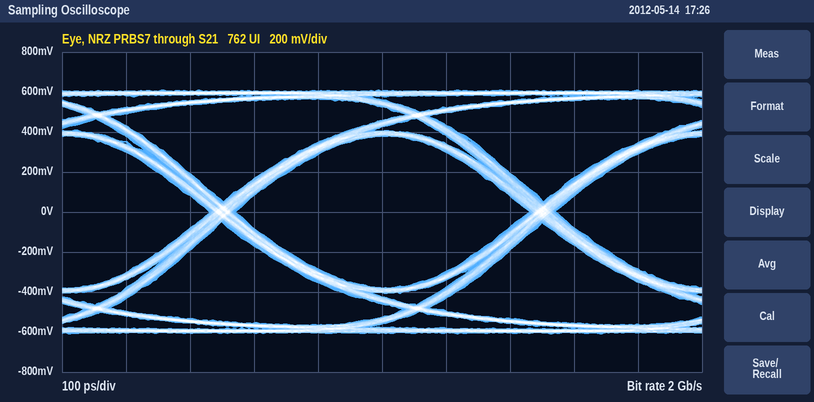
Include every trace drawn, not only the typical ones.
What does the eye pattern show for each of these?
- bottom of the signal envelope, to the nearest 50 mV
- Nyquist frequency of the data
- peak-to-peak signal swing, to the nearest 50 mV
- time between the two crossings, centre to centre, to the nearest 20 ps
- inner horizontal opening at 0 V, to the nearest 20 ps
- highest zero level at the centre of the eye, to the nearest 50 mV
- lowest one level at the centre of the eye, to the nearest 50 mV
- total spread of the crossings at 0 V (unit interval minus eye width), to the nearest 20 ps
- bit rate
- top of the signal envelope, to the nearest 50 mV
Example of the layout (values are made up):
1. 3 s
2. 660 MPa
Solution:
1. -600 mV
2. 1 GHz
3. 1.20 V
4. 500 ps
5. 460 ps
6. -400 mV
7. 400 mV
8. 40 ps
9. 2 Gb/s
10. 600 mV
